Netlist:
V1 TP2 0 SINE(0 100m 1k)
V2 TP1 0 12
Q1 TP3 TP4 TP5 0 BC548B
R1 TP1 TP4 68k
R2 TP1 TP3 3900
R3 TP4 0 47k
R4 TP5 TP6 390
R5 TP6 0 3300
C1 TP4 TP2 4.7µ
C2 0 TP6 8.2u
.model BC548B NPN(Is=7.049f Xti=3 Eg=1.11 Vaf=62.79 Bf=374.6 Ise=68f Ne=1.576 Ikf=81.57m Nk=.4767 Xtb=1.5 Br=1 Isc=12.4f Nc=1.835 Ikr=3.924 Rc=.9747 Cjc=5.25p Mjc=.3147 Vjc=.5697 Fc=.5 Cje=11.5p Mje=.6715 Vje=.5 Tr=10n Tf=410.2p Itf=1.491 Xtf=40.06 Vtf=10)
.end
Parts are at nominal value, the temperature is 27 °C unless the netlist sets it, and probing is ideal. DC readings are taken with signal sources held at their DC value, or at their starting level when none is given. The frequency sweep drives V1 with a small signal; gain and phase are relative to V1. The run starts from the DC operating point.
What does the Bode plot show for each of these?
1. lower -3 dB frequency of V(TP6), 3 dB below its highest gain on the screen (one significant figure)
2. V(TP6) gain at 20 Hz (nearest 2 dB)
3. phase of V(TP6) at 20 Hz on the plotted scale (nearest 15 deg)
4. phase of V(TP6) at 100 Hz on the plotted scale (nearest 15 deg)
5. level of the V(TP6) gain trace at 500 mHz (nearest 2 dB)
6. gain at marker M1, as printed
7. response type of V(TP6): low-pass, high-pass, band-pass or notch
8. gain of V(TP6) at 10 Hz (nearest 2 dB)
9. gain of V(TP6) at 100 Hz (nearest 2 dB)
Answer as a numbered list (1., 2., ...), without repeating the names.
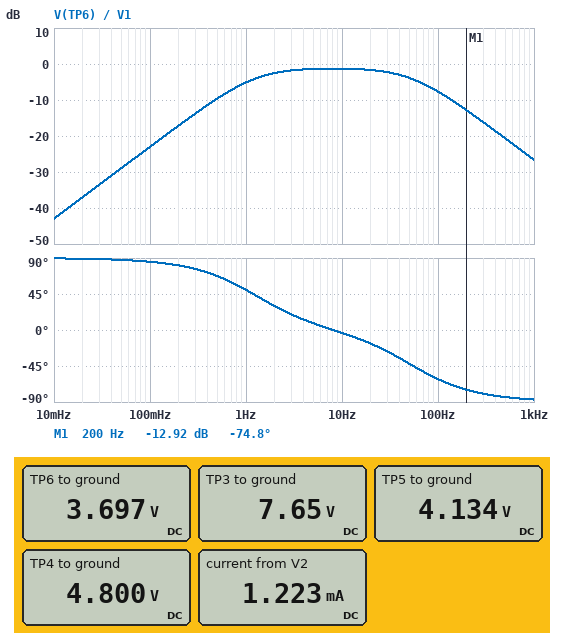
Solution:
1. 1 Hz
2. -2 dB
3. -15 deg
4. -60 deg
5. -10 dB
6. -12.92 dB
7. band-pass
8. -2 dB
9. -8 dB
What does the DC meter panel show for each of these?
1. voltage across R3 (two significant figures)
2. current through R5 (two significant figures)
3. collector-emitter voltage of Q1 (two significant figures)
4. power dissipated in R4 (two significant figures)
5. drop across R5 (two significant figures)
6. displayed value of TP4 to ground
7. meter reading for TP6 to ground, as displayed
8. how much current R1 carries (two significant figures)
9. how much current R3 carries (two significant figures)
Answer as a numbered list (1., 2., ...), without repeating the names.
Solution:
1. 4.8 V
2. 1.1 mA
3. 3.5 V
4. 490 µW
5. 3.7 V
6. 4.800 V
7. 3.697 V
8. 110 µA
9. 100 µA
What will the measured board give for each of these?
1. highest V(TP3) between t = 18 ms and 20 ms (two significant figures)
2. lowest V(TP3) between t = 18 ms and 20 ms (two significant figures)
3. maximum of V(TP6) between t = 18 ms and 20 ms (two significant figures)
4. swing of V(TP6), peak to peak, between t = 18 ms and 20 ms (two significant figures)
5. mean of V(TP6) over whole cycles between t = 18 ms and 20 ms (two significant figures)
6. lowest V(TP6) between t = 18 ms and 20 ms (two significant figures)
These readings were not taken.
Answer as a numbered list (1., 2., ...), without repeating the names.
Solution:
1. 8.6 V
2. 6.7 V
3. 3.7 V
4. 9.3 mV
5. 3.7 V
6. 3.7 V
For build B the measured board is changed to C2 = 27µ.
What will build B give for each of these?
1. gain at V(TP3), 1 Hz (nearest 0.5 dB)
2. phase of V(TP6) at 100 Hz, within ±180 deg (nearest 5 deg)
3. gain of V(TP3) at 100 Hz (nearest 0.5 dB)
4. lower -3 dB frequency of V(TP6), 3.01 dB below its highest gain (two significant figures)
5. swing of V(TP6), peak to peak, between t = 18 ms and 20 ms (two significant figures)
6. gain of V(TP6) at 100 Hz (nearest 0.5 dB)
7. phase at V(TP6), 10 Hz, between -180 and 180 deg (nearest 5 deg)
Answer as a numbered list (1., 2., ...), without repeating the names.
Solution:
1. -2.5 dB
2. -80 deg
3. 19.5 dB
4. 1.1 Hz
5. 2.9 mV
6. -17.0 dB
7. -25 deg
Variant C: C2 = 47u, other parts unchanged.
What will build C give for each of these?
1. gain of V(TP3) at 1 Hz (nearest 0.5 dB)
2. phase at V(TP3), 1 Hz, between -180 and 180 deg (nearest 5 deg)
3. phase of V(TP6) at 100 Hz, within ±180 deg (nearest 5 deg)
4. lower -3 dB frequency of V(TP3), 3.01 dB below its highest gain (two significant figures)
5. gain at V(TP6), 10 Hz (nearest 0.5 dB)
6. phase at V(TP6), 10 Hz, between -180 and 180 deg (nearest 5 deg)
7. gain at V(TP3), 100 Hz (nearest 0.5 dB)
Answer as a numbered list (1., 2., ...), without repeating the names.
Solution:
1. -1.0 dB
2. -90 deg
3. -85 deg
4. 9.5 Hz
5. -4.5 dB
6. -40 deg
7. 19.5 dB
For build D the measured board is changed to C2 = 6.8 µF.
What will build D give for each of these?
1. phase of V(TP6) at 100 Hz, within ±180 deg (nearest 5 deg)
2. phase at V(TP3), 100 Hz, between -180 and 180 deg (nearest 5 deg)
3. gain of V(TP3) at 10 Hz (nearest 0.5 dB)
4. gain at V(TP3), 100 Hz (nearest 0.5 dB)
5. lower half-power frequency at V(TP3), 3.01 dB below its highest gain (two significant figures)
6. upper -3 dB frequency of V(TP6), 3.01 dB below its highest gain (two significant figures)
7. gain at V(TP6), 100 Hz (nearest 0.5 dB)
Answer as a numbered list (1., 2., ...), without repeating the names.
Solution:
1. -55 deg
2. -150 deg
3. 5.0 dB
4. 18.0 dB
5. 63 Hz
6. 66 Hz
7. -6.5 dB
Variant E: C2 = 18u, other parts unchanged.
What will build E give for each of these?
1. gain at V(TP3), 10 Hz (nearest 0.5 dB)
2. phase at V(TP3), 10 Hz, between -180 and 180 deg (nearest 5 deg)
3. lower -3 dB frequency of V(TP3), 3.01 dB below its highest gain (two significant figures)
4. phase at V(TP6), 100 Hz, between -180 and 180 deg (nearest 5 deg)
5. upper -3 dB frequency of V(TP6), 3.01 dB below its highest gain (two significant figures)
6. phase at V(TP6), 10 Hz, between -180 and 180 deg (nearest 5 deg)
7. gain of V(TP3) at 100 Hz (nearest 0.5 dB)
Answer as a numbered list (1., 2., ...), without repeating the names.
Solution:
1. 11.5 dB
2. -120 deg
3. 24 Hz
4. -75 deg
5. 27 Hz
6. -15 deg
7. 19.0 dB
